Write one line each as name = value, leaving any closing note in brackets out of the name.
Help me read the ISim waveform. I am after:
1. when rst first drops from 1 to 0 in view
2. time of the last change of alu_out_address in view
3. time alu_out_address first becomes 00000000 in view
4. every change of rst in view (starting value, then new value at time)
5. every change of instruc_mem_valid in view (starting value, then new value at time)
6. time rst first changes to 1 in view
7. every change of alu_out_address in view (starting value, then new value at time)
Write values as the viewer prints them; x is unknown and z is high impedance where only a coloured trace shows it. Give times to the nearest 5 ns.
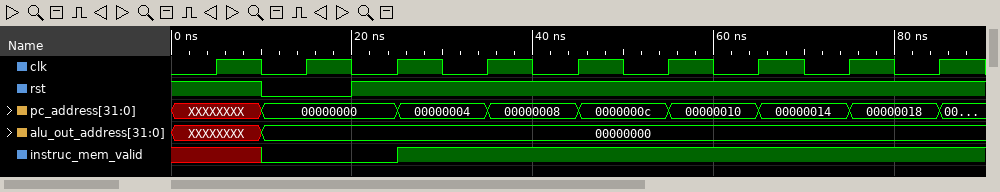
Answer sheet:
when rst first drops from 1 to 0 in view = 10 ns
time of the last change of alu_out_address in view = 10 ns
time alu_out_address first becomes 00000000 in view = 10 ns
every change of rst in view = 1, 0 at 10 ns, 1 at 20 ns
every change of instruc_mem_valid in view = x, 0 at 10 ns, 1 at 25 ns
time rst first changes to 1 in view = 20 ns
every change of alu_out_address in view = XXXXXXXX, 00000000 at 10 ns
